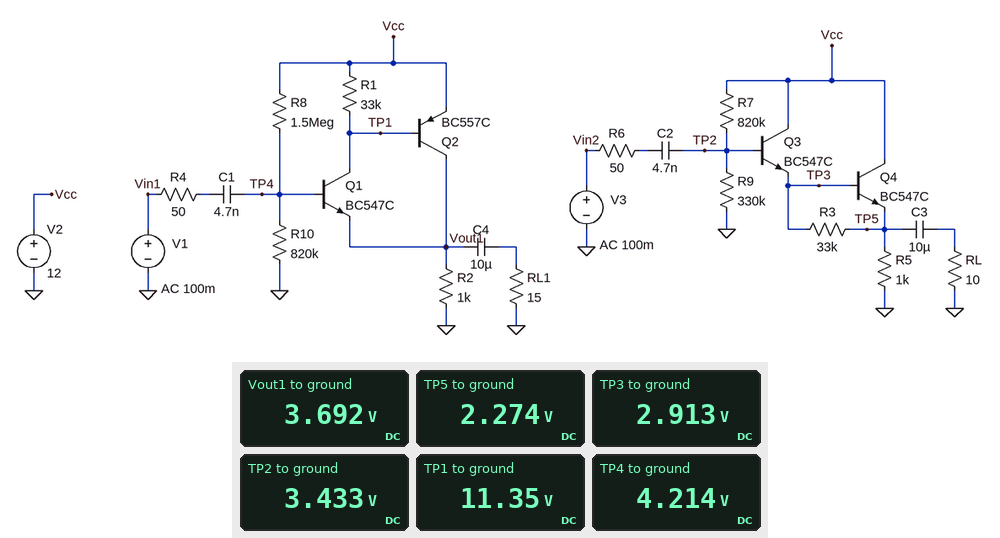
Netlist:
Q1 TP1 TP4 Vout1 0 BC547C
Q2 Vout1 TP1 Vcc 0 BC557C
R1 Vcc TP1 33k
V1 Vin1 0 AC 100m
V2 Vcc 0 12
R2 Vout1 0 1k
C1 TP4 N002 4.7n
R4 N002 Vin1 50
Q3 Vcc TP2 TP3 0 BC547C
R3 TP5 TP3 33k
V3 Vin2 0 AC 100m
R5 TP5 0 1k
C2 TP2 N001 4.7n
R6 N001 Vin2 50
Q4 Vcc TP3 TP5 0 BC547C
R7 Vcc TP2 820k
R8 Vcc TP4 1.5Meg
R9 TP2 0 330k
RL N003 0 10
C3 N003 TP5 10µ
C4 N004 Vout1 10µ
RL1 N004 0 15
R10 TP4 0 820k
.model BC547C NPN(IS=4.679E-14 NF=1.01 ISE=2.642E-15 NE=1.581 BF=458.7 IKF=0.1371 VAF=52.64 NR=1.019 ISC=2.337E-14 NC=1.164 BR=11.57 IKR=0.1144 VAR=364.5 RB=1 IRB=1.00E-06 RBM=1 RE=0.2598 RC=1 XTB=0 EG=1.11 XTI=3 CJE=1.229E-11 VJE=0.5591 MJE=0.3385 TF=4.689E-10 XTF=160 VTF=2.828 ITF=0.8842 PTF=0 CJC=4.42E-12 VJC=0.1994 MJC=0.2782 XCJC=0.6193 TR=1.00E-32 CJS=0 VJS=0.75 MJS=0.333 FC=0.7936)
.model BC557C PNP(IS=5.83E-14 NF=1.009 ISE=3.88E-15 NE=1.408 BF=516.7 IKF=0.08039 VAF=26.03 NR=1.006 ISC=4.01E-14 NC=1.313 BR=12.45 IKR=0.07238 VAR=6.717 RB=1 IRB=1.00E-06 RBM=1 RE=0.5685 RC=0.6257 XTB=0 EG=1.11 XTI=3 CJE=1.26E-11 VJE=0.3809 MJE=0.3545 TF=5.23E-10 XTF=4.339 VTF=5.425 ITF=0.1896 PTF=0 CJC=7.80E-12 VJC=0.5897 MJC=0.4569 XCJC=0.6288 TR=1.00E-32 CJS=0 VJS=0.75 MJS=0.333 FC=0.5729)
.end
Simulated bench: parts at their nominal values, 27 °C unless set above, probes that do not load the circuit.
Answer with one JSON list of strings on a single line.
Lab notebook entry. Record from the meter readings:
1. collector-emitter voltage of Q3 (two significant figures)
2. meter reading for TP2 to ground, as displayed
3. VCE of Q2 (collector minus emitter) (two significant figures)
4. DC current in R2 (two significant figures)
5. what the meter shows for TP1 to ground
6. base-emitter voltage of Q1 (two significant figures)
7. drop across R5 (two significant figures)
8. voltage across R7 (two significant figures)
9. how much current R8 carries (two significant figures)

["9.1 V", "3.433 V", "-8.3 V", "3.7 mA", "11.35 V", "520 mV", "2.3 V", "8.6 V", "5.2 µA"]
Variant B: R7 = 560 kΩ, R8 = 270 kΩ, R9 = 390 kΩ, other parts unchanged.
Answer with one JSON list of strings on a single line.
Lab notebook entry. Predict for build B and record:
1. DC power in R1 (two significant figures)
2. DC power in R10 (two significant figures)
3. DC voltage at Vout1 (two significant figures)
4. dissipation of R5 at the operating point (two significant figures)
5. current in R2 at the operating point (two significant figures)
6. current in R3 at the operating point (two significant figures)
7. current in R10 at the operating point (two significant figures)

["14 µW", "99 µW", "8.5 V", "14 mW", "8.5 mA", "20 µA", "11 µA"]
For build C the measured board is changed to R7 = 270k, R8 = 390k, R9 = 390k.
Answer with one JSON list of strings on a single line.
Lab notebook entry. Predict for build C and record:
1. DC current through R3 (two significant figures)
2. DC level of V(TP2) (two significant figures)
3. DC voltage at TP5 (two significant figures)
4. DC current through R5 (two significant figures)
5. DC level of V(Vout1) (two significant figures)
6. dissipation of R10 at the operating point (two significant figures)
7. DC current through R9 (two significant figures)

["20 µA", "7.1 V", "5.9 V", "5.9 mA", "7.6 V", "80 µW", "18 µA"]
